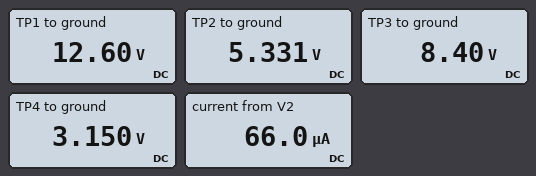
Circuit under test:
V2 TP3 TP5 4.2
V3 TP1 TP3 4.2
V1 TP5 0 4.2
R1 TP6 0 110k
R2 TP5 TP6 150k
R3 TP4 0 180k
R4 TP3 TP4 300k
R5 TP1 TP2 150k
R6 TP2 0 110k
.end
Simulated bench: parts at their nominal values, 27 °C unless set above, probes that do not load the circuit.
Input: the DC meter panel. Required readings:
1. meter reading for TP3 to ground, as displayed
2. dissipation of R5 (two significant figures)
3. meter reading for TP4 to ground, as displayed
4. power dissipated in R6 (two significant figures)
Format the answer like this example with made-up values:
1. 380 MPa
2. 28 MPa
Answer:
1. 8.40 V
2. 350 µW
3. 3.150 V
4. 260 µW
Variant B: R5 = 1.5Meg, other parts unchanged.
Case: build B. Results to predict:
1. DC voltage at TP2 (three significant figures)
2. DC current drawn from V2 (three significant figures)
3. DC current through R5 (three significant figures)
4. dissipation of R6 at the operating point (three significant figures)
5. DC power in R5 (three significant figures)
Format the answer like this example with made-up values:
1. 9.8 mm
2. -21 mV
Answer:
1. 861 mV
2. 25.3 µA
3. 7.83 µA
4. 6.74 µW
5. 91.9 µW
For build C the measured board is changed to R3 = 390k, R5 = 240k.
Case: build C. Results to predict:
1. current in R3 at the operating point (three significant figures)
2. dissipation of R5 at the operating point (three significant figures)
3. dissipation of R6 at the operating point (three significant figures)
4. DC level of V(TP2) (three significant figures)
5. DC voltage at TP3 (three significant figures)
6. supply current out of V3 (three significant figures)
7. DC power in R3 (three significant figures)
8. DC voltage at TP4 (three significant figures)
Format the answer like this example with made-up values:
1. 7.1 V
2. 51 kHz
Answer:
1. 12.2 µA
2. 311 µW
3. 143 µW
4. 3.96 V
5. 8.40 V
6. 36.0 µA
7. 57.8 µW
8. 4.75 V
